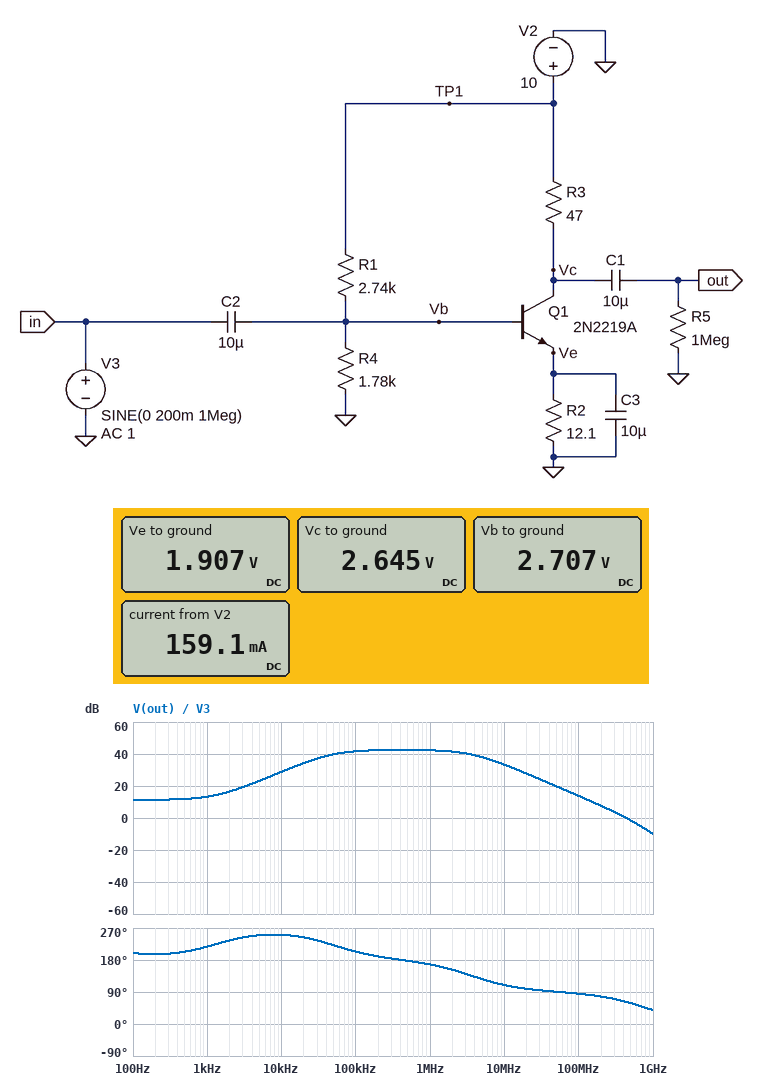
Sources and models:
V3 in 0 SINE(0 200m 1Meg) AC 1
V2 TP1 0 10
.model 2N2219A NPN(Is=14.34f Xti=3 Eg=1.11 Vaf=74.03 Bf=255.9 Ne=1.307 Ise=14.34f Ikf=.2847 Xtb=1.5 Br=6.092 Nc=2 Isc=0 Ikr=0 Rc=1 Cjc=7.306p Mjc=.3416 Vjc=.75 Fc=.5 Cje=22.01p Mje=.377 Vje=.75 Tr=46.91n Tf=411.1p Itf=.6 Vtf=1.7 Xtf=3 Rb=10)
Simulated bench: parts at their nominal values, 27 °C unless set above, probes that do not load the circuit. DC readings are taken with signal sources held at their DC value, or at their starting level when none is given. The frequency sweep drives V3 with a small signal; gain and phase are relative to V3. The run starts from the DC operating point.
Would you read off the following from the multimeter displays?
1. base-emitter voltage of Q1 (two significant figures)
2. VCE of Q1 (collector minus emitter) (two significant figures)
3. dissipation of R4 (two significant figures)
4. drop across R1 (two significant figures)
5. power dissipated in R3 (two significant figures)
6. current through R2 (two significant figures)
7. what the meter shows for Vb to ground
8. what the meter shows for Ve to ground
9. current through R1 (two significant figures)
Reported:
800 mV
740 mV
4.1 mW
7.3 V
1.2 W
160 mA
2.707 V
1.907 V
2.7 mA
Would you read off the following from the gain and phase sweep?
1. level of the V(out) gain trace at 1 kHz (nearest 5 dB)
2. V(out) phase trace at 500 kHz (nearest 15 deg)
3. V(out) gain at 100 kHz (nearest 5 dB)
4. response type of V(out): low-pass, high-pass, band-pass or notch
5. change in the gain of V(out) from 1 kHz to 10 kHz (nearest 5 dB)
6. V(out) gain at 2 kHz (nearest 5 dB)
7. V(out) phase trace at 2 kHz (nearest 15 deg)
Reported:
15 dB
180 deg
40 dB
band-pass
15 dB
15 dB
240 deg
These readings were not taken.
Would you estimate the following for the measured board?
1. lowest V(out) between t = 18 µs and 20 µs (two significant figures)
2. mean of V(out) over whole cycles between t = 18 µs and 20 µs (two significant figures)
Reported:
-570 mV
1.2 V
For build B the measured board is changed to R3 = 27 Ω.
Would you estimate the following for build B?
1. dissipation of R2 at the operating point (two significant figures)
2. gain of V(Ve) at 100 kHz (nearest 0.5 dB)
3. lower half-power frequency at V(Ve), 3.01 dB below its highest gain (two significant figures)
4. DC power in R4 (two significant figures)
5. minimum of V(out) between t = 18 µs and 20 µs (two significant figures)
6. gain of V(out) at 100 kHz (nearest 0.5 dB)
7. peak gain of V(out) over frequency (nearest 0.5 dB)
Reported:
310 mW
-7.0 dB
27 Hz
4.2 mW
-3.4 V
37.5 dB
38.5 dB
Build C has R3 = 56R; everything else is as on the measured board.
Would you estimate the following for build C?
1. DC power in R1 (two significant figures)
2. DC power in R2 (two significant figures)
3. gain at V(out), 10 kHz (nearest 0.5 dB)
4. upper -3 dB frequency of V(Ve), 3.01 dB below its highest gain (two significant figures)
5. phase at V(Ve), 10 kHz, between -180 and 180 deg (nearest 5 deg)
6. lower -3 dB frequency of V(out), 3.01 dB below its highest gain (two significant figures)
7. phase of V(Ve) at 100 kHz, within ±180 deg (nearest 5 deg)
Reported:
20 mW
250 mW
16.5 dB
6.9 kHz
-55 deg
5.9 kHz
-90 deg
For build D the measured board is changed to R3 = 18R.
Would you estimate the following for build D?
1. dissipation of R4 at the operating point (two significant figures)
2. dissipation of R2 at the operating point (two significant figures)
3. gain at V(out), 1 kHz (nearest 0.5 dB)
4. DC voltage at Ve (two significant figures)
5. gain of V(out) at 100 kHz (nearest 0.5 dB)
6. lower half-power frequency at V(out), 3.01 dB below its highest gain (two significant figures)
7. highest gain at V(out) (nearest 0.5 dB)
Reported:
4.3 mW
320 mW
5.0 dB
2.0 V
34.0 dB
52 kHz
35.0 dB
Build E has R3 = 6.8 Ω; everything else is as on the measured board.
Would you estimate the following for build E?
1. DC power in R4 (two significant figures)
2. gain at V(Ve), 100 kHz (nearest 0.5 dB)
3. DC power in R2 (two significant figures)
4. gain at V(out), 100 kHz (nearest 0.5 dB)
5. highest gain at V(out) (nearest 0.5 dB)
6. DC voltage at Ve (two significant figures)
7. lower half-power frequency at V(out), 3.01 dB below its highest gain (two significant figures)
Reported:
4.3 mW
-6.5 dB
320 mW
26.0 dB
27.0 dB
2.0 V
54 kHz
